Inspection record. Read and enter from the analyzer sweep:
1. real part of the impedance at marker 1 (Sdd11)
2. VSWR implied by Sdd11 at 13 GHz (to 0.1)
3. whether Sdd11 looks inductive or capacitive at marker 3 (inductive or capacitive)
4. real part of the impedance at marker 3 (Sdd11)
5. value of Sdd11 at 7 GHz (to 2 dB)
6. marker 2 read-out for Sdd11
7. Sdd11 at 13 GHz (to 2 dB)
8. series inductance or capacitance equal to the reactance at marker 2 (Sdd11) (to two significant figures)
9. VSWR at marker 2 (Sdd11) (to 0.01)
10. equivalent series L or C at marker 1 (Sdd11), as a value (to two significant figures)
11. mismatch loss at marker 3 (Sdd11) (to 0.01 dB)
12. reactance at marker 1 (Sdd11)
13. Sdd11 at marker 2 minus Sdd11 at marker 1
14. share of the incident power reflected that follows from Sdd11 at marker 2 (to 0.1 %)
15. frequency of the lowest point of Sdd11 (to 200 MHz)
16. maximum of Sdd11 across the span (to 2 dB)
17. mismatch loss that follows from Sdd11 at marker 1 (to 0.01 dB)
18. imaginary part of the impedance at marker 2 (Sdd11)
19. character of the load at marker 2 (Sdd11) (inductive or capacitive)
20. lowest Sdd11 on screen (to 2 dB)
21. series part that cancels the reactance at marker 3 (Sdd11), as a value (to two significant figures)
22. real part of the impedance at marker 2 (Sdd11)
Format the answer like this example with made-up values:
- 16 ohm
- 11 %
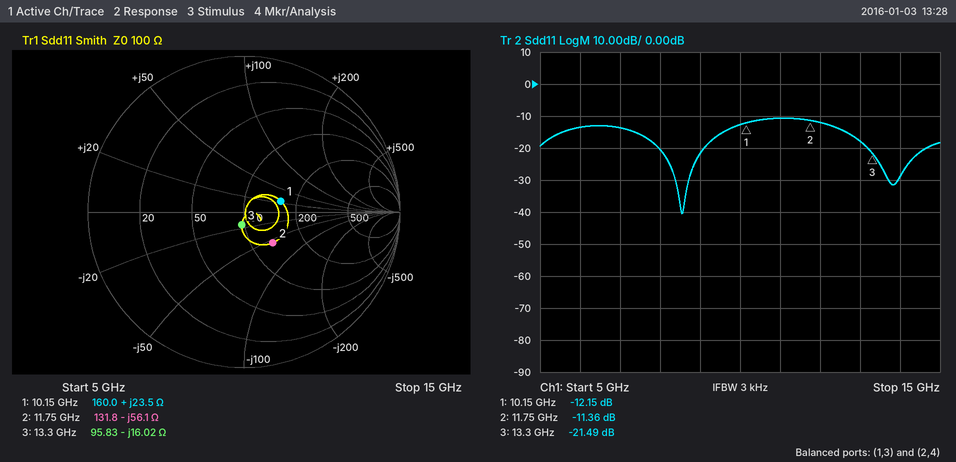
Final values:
- 160.0 Ω
- 1.3
- capacitive
- 95.83 Ω
- -14 dB
- -11.36 dB
- -18 dB
- 240 fF
- 1.74
- 370 pH
- 0.03 dB
- +23.5 Ω
- 0.79 dB
- 7.3 %
- 8.6 GHz
- -10 dB
- 0.27 dB
- -56.1 Ω
- capacitive
- -40 dB
- 190 pH
- 131.8 Ω
